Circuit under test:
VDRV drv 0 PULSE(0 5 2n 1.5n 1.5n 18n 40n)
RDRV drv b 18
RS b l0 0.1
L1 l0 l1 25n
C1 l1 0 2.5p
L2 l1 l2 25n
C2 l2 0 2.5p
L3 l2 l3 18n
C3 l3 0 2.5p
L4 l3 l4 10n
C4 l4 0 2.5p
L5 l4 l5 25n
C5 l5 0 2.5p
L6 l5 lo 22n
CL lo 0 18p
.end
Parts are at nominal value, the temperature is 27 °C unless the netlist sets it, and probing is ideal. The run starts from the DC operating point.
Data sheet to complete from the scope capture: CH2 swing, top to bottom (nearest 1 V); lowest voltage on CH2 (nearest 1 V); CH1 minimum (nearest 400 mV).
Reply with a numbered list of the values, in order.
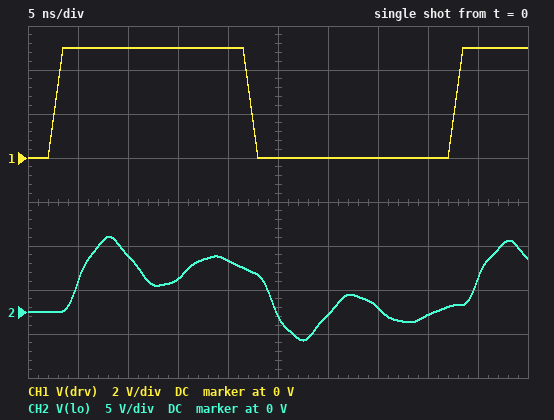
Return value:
1. 12 V
2. -3 V
3. 0 V
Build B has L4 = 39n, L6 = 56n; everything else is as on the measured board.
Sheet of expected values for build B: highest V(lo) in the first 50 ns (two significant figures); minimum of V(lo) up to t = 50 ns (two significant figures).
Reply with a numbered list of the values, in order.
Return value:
1. 9.8 V
2. -5.0 V
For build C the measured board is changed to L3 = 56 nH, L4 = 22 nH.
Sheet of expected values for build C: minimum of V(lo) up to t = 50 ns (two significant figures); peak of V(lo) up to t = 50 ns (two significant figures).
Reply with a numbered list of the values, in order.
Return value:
1. -4.8 V
2. 9.8 V
